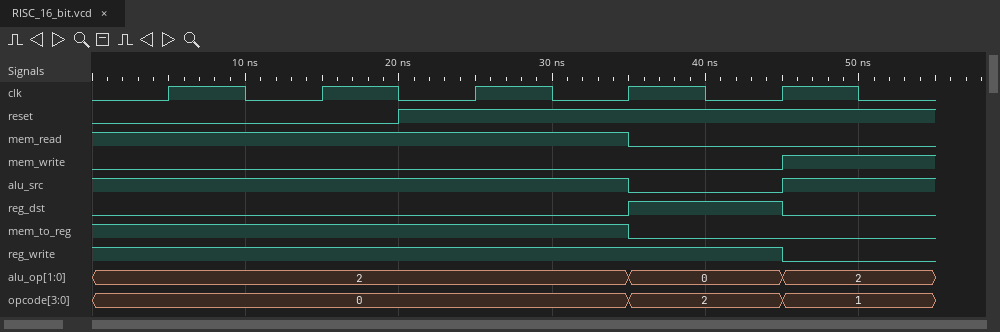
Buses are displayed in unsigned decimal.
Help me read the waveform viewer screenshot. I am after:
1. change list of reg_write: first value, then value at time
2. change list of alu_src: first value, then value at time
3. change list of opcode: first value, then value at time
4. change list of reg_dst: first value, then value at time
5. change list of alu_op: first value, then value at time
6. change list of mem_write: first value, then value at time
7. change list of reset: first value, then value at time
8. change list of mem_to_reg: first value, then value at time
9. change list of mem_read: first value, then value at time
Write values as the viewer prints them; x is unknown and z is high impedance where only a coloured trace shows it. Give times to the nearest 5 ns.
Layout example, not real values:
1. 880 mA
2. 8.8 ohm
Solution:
1. 1, 0 at 45 ns
2. 1, 0 at 35 ns, 1 at 45 ns
3. 0, 2 at 35 ns, 1 at 45 ns
4. 0, 1 at 35 ns, 0 at 45 ns
5. 2, 0 at 35 ns, 2 at 45 ns
6. 0, 1 at 45 ns
7. 0, 1 at 20 ns
8. 1, 0 at 35 ns
9. 1, 0 at 35 ns
